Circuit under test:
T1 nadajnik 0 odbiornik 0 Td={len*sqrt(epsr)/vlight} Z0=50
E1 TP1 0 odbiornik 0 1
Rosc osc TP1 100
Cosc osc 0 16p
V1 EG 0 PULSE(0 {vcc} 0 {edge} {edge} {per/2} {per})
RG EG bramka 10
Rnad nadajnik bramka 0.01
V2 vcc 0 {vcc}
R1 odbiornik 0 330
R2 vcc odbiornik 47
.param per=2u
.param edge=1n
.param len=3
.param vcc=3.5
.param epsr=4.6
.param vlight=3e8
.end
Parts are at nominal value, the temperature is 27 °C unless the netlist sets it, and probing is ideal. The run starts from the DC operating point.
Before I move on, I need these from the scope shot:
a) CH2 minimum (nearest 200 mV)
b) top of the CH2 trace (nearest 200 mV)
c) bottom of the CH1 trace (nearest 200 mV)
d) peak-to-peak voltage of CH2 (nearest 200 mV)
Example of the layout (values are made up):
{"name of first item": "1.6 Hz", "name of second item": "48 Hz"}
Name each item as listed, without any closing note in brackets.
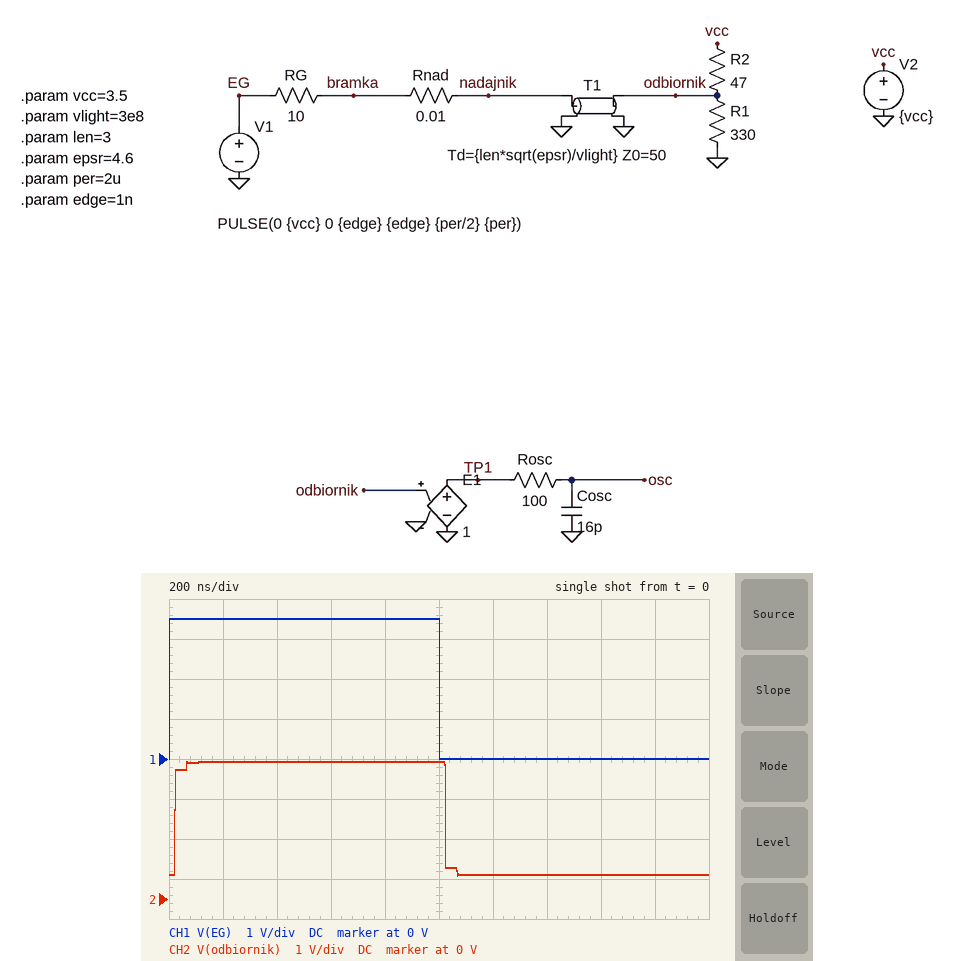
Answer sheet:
{"CH2 minimum": "600 mV", "top of the CH2 trace": "3.4 V", "bottom of the CH1 trace": "0 V", "peak-to-peak voltage of CH2": "2.8 V"}
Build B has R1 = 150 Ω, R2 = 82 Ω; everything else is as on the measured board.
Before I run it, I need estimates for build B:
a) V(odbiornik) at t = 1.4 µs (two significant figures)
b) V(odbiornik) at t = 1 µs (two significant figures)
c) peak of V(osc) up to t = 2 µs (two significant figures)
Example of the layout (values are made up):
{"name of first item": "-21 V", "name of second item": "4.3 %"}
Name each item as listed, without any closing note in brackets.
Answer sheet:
{"V(odbiornik) at t = 1.4 µs": "360 mV", "V(odbiornik) at t = 1 µs": "3.3 V", "peak of V(osc) up to t = 2 µs": "3.4 V"}
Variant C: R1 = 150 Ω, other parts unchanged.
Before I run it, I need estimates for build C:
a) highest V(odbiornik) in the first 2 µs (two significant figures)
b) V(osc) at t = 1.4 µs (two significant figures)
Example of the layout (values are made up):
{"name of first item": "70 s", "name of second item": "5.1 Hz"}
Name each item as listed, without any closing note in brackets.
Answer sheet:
{"highest V(odbiornik) in the first 2 µs": "3.3 V", "V(osc) at t = 1.4 µs": "580 mV"}
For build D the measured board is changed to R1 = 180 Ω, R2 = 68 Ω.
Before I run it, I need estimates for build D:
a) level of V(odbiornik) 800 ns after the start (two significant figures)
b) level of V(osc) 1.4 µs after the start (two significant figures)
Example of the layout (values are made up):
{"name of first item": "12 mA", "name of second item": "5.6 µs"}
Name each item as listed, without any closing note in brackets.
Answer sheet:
{"level of V(odbiornik) 800 ns after the start": "3.3 V", "level of V(osc) 1.4 µs after the start": "430 mV"}
